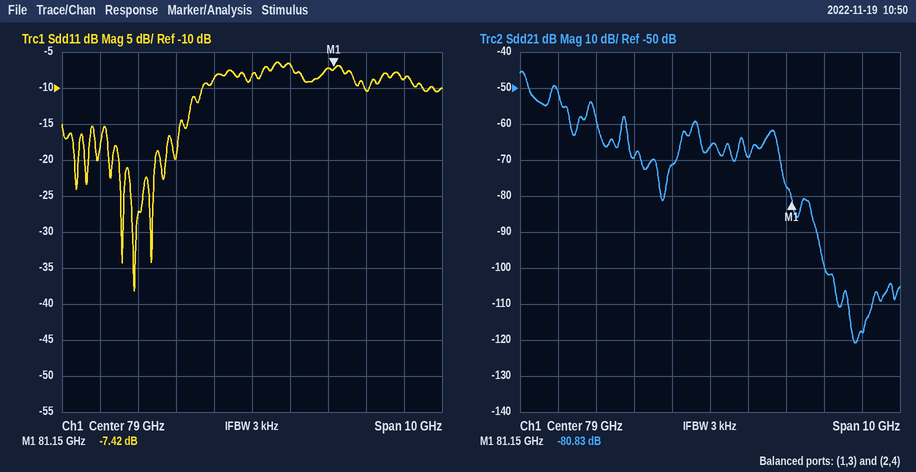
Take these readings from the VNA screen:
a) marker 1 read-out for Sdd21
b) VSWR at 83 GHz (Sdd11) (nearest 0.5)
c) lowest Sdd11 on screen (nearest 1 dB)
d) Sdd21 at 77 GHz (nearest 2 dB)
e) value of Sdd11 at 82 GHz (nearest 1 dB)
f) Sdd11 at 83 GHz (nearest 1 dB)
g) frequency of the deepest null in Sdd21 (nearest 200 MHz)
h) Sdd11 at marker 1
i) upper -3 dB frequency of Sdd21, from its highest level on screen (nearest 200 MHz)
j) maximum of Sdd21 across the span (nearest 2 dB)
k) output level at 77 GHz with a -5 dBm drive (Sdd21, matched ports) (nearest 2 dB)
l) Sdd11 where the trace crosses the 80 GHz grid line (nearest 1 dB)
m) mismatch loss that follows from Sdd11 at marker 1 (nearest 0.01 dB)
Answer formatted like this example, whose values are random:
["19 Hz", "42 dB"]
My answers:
["-80.83 dB", "2.0", "-38 dB", "-70 dB", "-10 dB", "-9 dB", "82.8 GHz", "-7.42 dB", "74.2 GHz", "-46 dB", "-74 dBm", "-7 dB", "0.87 dB"]
